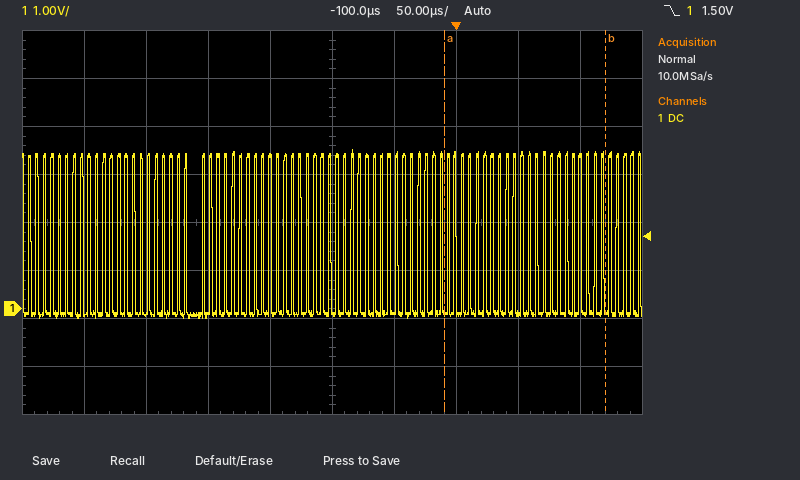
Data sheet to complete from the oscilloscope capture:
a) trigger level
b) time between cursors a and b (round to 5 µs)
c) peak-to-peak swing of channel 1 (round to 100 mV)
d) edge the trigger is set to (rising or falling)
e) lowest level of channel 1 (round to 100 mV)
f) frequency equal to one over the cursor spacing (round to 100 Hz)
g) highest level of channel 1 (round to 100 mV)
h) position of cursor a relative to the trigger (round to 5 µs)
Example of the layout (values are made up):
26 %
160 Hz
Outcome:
1.50 V
130 µs
3.5 V
falling
-200 mV
7.7 kHz
3.3 V
-10 µs
